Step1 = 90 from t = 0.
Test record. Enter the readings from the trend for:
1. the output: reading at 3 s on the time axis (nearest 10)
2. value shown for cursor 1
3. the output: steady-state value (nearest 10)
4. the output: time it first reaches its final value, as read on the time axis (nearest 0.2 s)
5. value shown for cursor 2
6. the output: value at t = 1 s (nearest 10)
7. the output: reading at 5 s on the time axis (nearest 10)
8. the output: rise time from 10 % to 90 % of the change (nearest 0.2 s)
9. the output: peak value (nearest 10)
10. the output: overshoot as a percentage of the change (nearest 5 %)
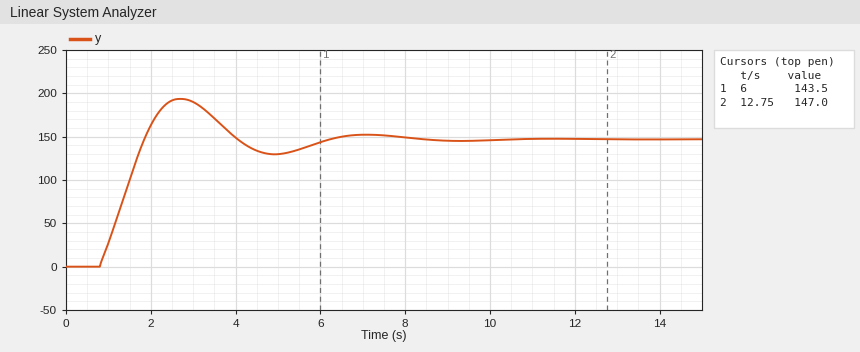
190
143.5
150
1.8 s
147.0
30
130
0.8 s
190
30 %
